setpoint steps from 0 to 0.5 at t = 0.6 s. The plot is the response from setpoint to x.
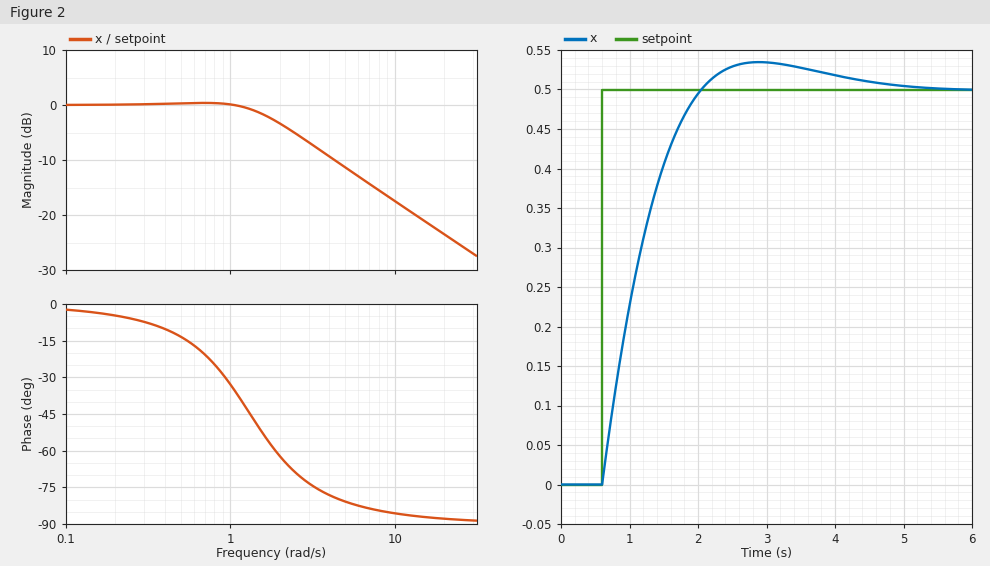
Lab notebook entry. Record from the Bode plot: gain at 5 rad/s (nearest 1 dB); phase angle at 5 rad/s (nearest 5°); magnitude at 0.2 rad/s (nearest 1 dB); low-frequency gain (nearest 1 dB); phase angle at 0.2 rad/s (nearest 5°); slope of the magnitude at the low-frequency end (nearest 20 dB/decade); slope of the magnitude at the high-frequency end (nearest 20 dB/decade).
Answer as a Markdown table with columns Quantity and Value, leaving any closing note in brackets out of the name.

| Quantity | Value |
|---|---|
| gain at 5 rad/s | -11 dB |
| phase angle at 5 rad/s | -80° |
| magnitude at 0.2 rad/s | 0 dB |
| low-frequency gain | 0 dB |
| phase angle at 0.2 rad/s | -5° |
| slope of the magnitude at the low-frequency end | 0 dB/decade |
| slope of the magnitude at the high-frequency end | -20 dB/decade |
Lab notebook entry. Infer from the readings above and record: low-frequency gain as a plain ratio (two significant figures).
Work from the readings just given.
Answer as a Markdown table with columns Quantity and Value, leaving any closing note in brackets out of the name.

| Quantity | Value |
|---|---|
| low-frequency gain as a plain ratio | 1.0 |
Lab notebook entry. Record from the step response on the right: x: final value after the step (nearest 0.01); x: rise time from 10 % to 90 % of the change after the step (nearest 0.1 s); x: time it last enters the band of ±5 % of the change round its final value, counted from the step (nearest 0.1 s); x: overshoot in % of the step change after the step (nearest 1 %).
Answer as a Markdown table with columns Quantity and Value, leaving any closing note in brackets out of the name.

| Quantity | Value |
|---|---|
| x: final value after the step | 0.50 |
| x: rise time from 10 % to 90 % of the change after the step | 1.0 s |
| x: time it last enters the band of ±5 % of the change round its final value, counted from the step | 3.0 s |
| x: overshoot in % of the step change after the step | 7 % |
